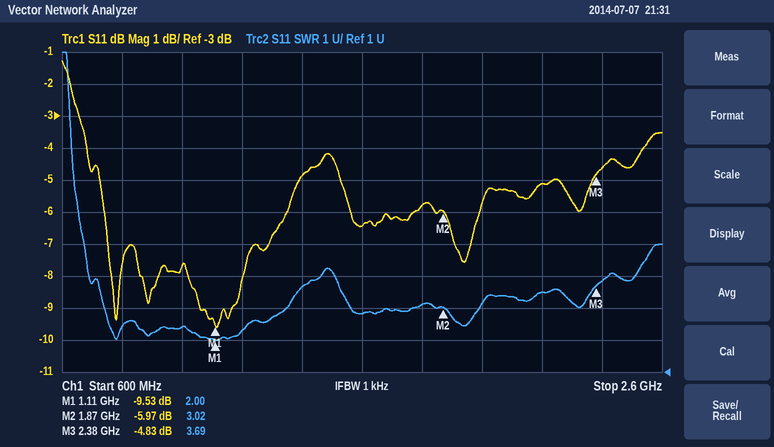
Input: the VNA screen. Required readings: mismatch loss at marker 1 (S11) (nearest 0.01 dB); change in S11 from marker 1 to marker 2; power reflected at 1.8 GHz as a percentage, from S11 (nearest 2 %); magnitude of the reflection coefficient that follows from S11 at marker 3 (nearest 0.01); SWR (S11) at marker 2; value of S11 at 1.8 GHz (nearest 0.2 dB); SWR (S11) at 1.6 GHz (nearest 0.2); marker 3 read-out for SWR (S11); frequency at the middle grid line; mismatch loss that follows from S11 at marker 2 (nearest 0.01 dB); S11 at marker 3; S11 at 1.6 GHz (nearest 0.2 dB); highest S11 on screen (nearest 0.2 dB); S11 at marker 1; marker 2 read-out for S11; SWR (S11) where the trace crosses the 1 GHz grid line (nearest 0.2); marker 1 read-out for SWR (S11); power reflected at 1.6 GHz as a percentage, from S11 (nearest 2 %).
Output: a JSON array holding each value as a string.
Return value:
["0.51 dB", "3.56 dB", "26 %", "0.57", "3.02", "-5.8 dB", "2.8", "3.69", "1.6 GHz", "1.27 dB", "-4.83 dB", "-6.4 dB", "-1.2 dB", "-9.53 dB", "-5.97 dB", "2.4", "2.00", "22 %"]
